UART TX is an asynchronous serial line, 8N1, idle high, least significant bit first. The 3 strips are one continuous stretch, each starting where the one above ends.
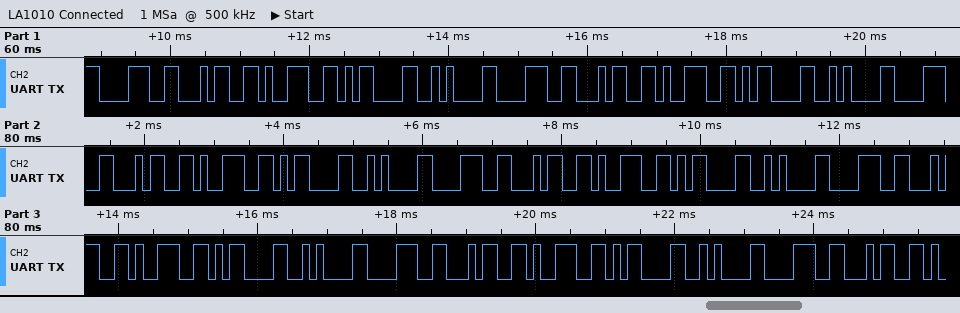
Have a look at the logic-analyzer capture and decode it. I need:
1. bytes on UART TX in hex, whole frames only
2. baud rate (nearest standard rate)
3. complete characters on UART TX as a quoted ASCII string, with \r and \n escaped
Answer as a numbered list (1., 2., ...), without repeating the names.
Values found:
1. 38 34 39 0D 0A 38 34 39 0D 0A 38 34 39 0D 0A 38 34 39 0D 0A 38 34 39 0D 0A 38 34 39 0D 0A 38 34
2. 9600 baud
3. "849\r\n849\r\n849\r\n849\r\n849\r\n849\r\n84"
